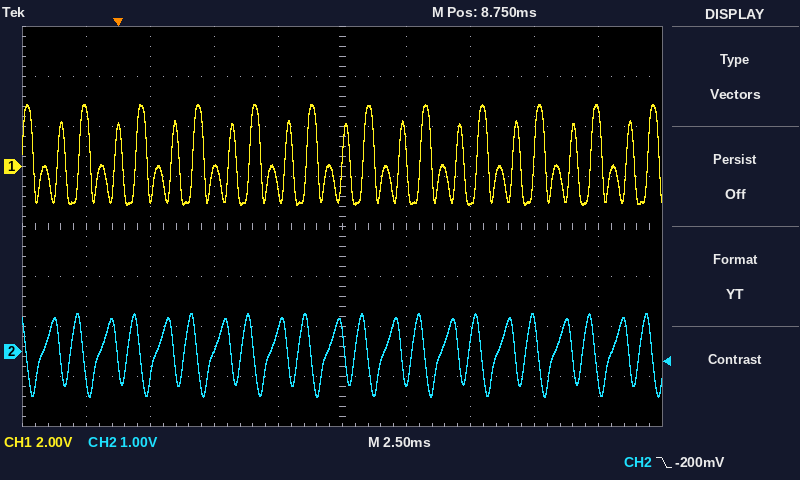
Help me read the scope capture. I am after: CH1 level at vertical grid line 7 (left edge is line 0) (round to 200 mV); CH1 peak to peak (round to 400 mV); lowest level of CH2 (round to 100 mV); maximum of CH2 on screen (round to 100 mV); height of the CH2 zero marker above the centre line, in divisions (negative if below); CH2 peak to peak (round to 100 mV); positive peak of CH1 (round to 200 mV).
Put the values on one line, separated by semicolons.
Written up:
-1.4 V; 4.0 V; -900 mV; 800 mV; -2.5 div; 1.7 V; 2.4 V
